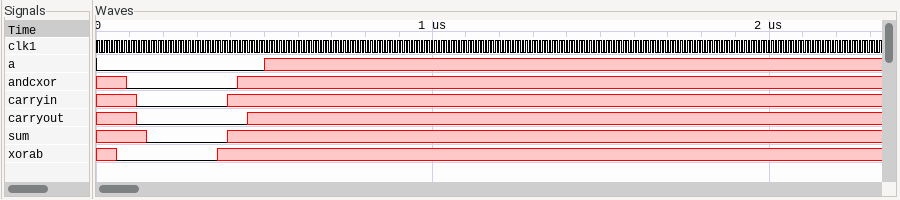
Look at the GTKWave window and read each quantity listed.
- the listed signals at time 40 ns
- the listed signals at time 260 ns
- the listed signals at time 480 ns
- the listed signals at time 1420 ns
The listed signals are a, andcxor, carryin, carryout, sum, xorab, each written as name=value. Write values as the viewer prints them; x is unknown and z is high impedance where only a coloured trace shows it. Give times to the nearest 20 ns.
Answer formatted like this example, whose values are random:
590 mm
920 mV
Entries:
a=0, andcxor=x, carryin=x, carryout=x, sum=x, xorab=x
a=0, andcxor=0, carryin=0, carryout=0, sum=0, xorab=0
a=0, andcxor=x, carryin=x, carryout=x, sum=x, xorab=x
a=x, andcxor=x, carryin=x, carryout=x, sum=x, xorab=x
